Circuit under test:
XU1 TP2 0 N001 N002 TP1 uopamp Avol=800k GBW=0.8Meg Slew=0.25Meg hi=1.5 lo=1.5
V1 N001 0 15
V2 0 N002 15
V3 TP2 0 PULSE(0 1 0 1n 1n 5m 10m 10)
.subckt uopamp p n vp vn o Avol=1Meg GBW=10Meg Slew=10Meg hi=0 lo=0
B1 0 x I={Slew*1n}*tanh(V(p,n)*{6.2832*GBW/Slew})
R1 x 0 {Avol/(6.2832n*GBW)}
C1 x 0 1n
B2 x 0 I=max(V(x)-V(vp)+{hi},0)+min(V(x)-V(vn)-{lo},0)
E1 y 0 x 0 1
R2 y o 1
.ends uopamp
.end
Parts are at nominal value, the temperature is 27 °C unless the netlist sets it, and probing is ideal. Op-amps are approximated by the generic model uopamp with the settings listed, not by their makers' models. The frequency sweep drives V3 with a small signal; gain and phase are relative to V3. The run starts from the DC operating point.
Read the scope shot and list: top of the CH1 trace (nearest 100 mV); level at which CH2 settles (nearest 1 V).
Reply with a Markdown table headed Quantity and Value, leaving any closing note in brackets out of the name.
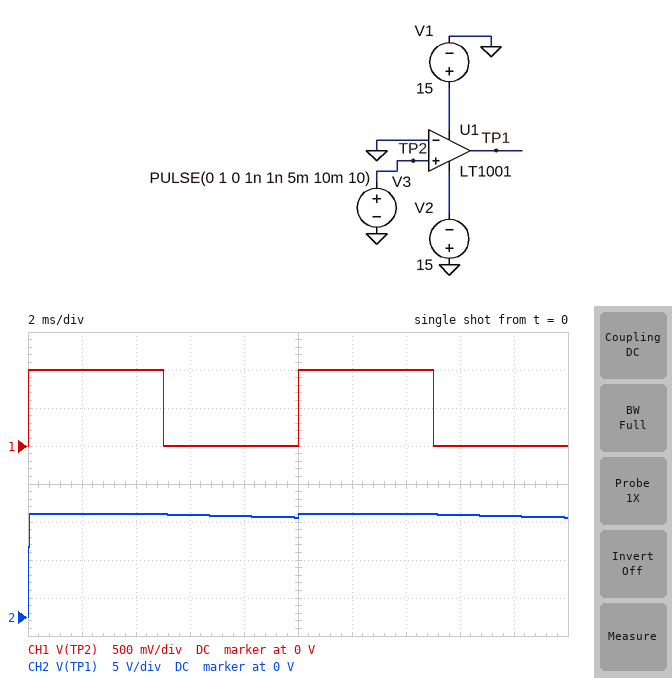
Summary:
| Quantity | Value |
|---|---|
| top of the CH1 trace | 1.0 V |
| level at which CH2 settles | 13 V |
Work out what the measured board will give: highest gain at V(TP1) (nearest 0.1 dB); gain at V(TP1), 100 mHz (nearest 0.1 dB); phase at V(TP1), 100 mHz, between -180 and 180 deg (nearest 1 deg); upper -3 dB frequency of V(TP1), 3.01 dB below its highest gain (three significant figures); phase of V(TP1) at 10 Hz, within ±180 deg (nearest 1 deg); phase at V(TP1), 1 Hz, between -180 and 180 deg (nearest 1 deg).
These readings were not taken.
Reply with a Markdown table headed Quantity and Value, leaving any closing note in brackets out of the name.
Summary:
| Quantity | Value |
|---|---|
| highest gain at V(TP1) | 118.1 dB |
| gain at V(TP1), 100 mHz | 118.0 dB |
| phase at V(TP1), 100 mHz, between -180 and 180 deg | -6 deg |
| upper -3 dB frequency of V(TP1), 3.01 dB below its highest gain | 1.00 Hz |
| phase of V(TP1) at 10 Hz, within ±180 deg | -84 deg |
| phase at V(TP1), 1 Hz, between -180 and 180 deg | -45 deg |
